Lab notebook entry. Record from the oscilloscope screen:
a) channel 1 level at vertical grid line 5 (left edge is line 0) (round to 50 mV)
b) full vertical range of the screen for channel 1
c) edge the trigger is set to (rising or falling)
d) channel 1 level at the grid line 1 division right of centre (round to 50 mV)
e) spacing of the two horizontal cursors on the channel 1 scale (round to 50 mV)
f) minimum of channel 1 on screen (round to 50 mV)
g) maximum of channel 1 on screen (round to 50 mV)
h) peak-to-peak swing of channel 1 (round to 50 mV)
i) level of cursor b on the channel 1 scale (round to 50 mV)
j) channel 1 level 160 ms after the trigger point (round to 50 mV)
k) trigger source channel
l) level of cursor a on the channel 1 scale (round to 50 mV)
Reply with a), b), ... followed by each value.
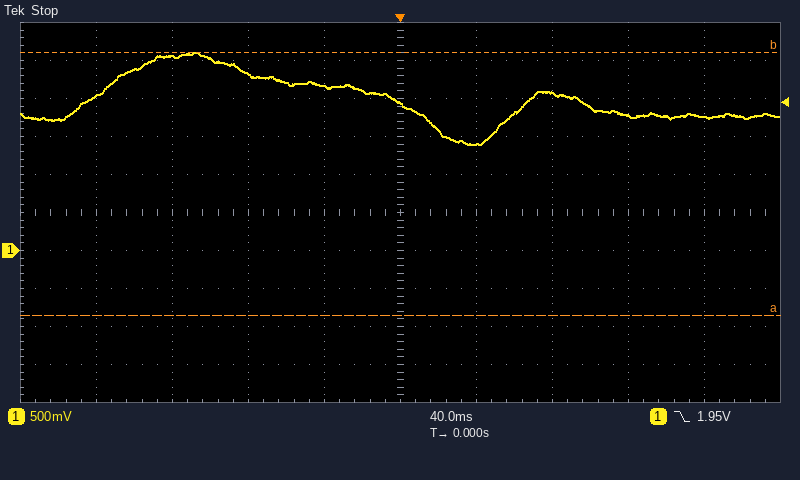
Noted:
a) 1.95 V
b) 5 V
c) falling
d) 1.40 V
e) 3.45 V
f) 1.40 V
g) 2.60 V
h) 1.20 V
i) 2.60 V
j) 1.75 V
k) channel 1
l) -850 mV
